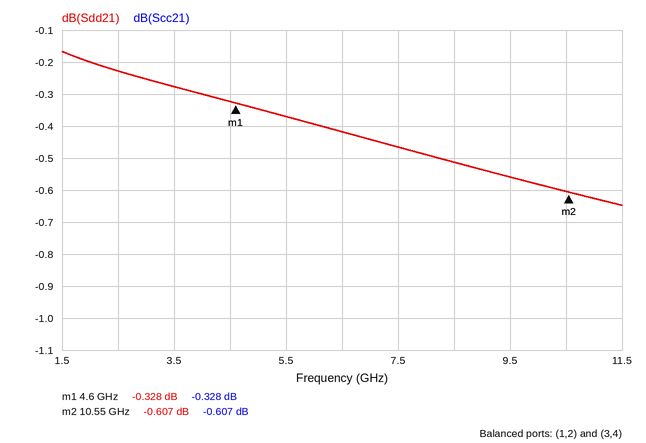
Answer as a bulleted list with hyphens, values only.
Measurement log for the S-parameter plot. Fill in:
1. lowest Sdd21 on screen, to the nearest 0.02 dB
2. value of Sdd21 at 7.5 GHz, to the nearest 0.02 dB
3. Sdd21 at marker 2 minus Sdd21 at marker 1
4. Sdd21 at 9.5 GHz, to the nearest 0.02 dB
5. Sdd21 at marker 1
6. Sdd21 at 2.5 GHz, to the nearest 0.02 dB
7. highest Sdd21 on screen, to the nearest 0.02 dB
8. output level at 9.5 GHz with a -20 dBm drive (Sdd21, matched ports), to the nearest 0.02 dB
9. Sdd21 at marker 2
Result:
- -0.64 dB
- -0.46 dB
- -0.279 dB
- -0.56 dB
- -0.328 dB
- -0.22 dB
- -0.16 dB
- -20.56 dBm
- -0.607 dB
